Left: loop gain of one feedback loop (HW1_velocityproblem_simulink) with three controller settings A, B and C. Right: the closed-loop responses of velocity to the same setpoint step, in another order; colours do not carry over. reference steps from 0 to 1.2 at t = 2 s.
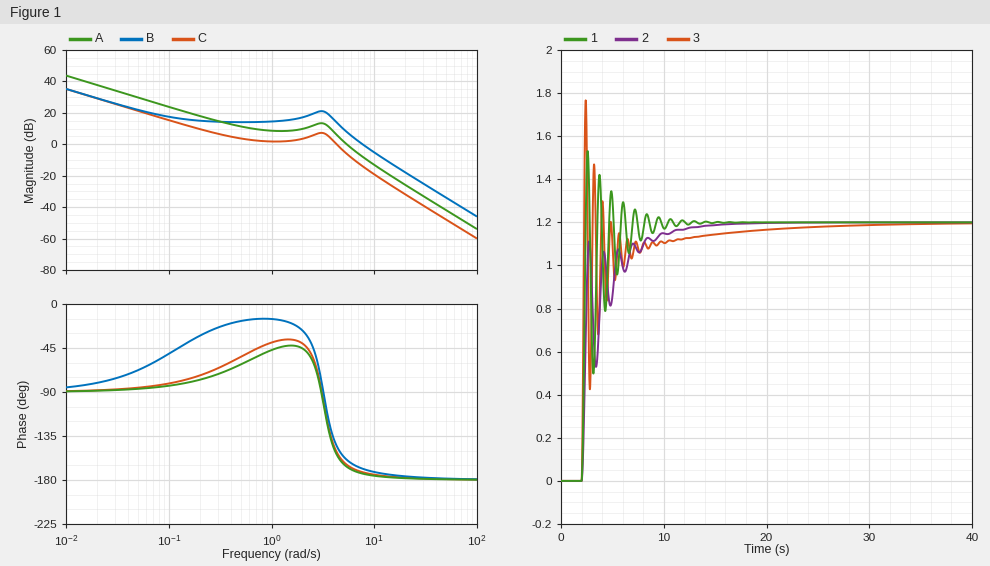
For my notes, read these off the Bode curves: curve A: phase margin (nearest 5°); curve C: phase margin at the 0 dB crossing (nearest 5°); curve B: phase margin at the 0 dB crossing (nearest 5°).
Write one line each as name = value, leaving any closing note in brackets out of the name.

curve A: phase margin = 15°
curve C: phase margin at the 0 dB crossing = 30°
curve B: phase margin at the 0 dB crossing = 10°
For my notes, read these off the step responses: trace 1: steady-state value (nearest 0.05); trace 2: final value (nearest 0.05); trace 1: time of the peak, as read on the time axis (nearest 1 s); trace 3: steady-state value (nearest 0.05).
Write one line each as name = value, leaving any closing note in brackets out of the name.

trace 1: steady-state value = 1.20
trace 2: final value = 1.20
trace 1: time of the peak, as read on the time axis = 3 s
trace 3: steady-state value = 1.20
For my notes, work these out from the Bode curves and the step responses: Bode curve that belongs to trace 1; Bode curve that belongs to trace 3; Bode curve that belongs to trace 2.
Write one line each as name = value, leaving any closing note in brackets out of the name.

Bode curve that belongs to trace 1 = A
Bode curve that belongs to trace 3 = B
Bode curve that belongs to trace 2 = C
